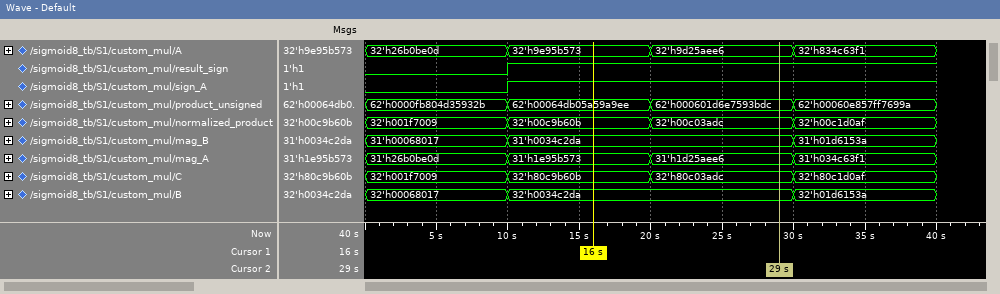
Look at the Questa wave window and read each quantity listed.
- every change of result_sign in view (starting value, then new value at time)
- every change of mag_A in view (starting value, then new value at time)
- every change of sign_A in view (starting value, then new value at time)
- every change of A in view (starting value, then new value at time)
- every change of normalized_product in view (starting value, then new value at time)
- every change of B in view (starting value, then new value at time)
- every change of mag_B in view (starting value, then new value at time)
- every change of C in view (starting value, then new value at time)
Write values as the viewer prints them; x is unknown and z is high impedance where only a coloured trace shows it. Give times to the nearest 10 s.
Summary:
0, 1 at 10 s
31'h26b0be0d, 31'h1e95b573 at 10 s, 31'h1d25aee6 at 20 s, 31'h034c63f1 at 30 s
0, 1 at 10 s
32'h26b0be0d, 32'h9e95b573 at 10 s, 32'h9d25aee6 at 20 s, 32'h834c63f1 at 30 s
32'h001f7009, 32'h00c9b60b at 10 s, 32'h00c03adc at 20 s, 32'h00c1d0af at 30 s
32'h00068017, 32'h0034c2da at 10 s, 32'h01d6153a at 30 s
31'h00068017, 31'h0034c2da at 10 s, 31'h01d6153a at 30 s
32'h001f7009, 32'h80c9b60b at 10 s, 32'h80c03adc at 20 s, 32'h80c1d0af at 30 s
